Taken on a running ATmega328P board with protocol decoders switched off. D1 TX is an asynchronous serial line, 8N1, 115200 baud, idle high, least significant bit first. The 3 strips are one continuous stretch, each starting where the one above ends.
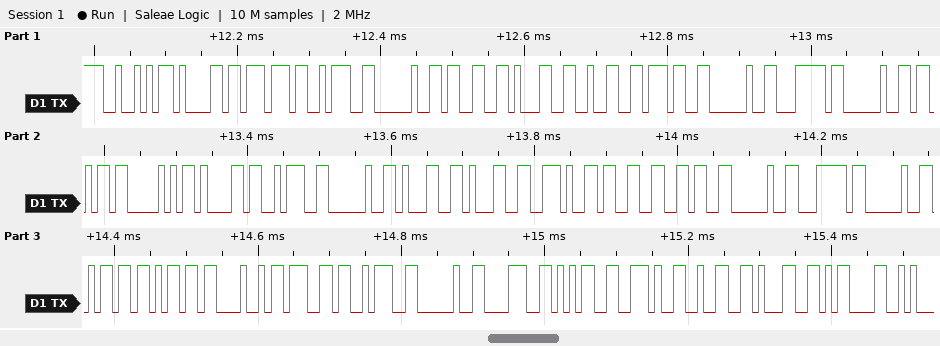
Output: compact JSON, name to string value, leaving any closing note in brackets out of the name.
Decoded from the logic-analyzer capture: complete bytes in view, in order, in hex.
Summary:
{"complete bytes in view, in order, in hex": "0x52 0x61 0x77 0x3A 0x20 0x33 0x31 0x32 0x37 0x20 0x7C 0x20 0x6B 0x50 0x61 0x3A 0x20 0x31 0x31 0x2E 0x33 0x36 0x20 0x7C 0x20 0x6D 0x6D 0x48 0x67 0x3A 0x20 0x38 0x35 0x2E 0x32 0x31 0x0D"}
